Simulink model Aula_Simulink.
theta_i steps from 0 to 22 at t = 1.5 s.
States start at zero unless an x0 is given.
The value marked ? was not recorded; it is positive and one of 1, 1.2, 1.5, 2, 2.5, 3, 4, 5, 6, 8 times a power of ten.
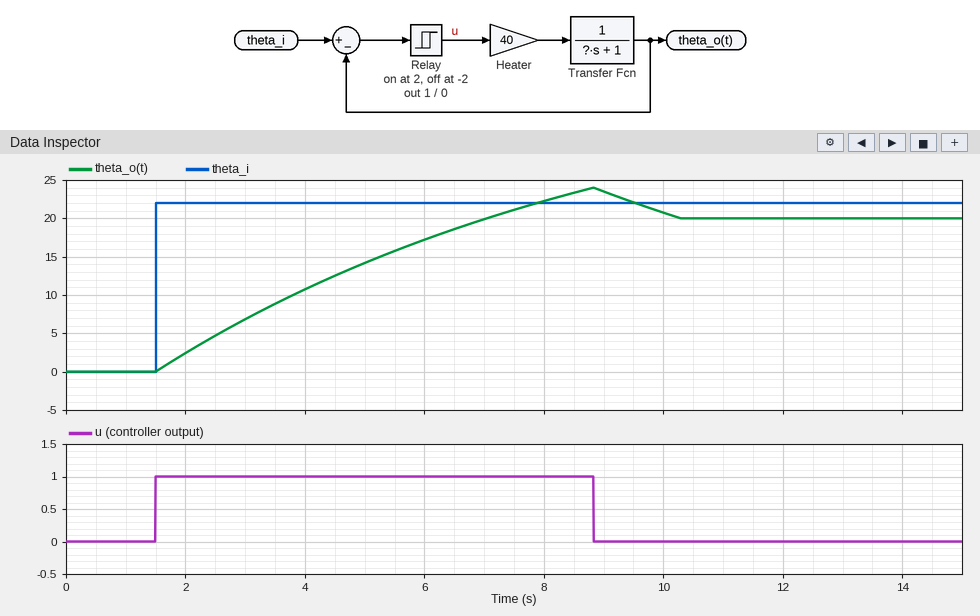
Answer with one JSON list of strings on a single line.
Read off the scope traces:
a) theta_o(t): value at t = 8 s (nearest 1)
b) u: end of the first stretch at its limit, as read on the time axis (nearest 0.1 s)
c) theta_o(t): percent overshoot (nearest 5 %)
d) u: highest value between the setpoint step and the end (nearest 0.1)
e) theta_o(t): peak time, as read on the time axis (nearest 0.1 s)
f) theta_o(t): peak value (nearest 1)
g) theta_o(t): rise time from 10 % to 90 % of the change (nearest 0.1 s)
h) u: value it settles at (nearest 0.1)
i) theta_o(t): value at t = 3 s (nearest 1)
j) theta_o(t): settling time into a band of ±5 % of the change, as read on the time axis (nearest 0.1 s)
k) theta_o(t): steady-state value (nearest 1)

["22", "8.8 s", "20 %", "1.0", "8.8 s", "24", "4.4 s", "0.0", "7", "9.9 s", "20"]
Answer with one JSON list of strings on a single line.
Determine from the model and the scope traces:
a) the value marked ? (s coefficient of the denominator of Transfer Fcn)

["8"]
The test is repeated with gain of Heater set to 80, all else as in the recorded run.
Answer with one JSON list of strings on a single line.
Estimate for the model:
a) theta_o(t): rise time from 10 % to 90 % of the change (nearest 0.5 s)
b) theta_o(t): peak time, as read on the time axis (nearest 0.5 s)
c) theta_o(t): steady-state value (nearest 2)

["2.0 s", "4.5 s", "20"]
